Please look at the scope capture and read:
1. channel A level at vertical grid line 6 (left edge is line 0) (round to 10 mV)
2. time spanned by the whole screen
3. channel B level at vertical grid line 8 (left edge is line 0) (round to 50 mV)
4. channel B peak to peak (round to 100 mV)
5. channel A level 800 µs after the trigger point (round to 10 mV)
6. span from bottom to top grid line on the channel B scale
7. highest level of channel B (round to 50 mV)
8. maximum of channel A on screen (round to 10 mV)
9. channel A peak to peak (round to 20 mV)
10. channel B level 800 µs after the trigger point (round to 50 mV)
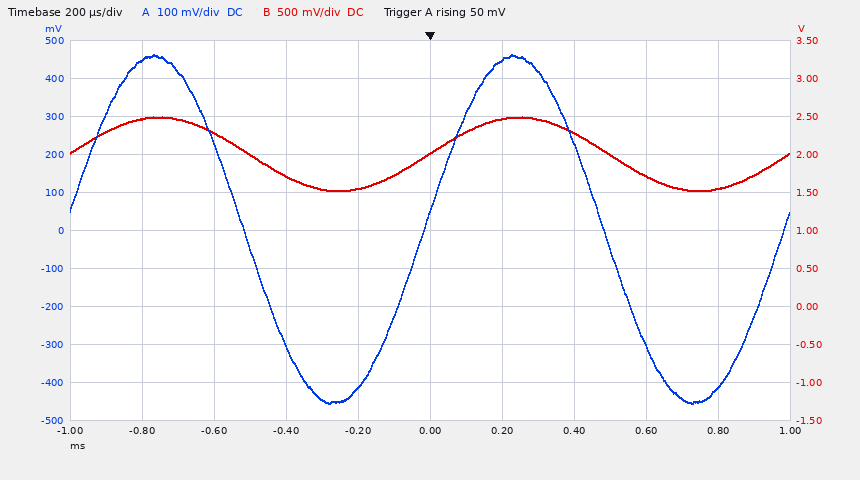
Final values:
450 mV
2 ms
1.70 V
1.00 V
-410 mV
5 V
2.50 V
460 mV
920 mV
1.55 V
